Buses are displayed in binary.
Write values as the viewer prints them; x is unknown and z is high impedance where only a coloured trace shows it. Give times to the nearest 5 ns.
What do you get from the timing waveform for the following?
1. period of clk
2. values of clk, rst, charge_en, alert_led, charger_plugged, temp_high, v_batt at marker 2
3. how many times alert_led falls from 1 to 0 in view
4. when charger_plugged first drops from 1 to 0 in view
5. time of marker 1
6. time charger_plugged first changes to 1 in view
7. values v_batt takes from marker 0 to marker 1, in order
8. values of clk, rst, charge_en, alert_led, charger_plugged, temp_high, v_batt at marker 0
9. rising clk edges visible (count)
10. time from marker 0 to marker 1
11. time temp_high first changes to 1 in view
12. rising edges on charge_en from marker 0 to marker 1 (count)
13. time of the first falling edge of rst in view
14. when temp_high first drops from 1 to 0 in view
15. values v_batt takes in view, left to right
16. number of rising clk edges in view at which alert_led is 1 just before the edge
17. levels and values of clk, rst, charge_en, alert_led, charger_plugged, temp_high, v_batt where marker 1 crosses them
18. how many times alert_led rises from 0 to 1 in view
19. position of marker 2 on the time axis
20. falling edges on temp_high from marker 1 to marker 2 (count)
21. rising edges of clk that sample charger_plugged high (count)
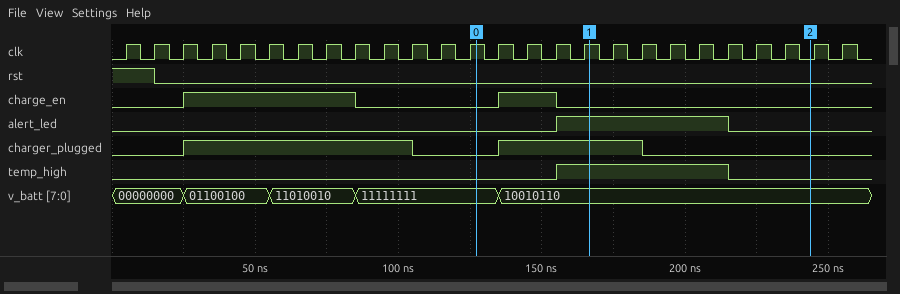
10 ns
clk=0, rst=0, charge_en=0, alert_led=0, charger_plugged=0, temp_high=0, v_batt=10010110
1
105 ns
165 ns
25 ns
11111111, 10010110
clk=1, rst=0, charge_en=0, alert_led=0, charger_plugged=0, temp_high=0, v_batt=11111111
26
40 ns
155 ns
1
15 ns
215 ns
00000000, 01100100, 11010010, 11111111, 10010110
6
clk=1, rst=0, charge_en=0, alert_led=1, charger_plugged=1, temp_high=1, v_batt=10010110
1
245 ns
1
13
